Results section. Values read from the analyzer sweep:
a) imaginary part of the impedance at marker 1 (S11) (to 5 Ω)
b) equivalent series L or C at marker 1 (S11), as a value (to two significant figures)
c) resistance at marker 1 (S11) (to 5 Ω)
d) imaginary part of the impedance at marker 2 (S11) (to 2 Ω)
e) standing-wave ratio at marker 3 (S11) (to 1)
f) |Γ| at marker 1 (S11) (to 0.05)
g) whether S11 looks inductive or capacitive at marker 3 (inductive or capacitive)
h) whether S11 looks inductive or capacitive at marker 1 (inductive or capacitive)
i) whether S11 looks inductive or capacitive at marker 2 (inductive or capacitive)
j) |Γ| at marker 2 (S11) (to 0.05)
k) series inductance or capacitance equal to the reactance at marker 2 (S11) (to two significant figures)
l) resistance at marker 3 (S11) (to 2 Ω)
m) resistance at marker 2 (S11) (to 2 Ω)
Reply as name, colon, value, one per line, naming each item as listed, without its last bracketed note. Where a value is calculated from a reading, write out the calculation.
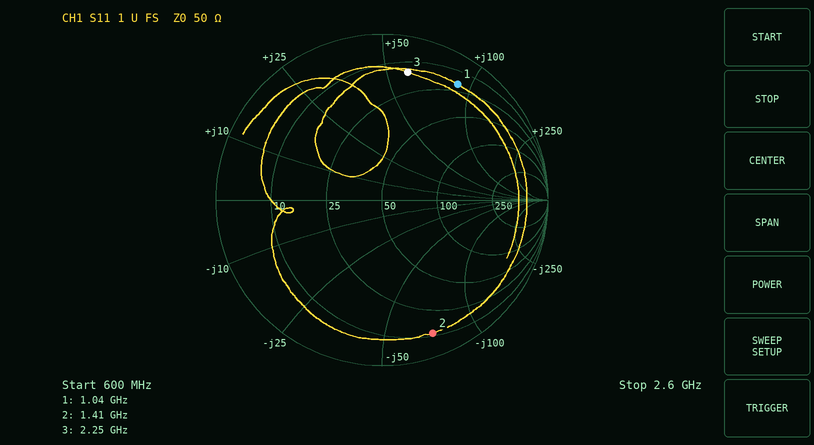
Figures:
imaginary part of the impedance at marker 1 (S11): +90 Ω
equivalent series L or C at marker 1 (S11), as a value: L = 90 Ω/(2π × 1.04 GHz) ≈ 14 nH
resistance at marker 1 (S11): 20 Ω
imaginary part of the impedance at marker 2 (S11): -72 Ω
standing-wave ratio at marker 3 (S11): 8
|Γ| at marker 1 (S11): 0.85
whether S11 looks inductive or capacitive at marker 3: inductive
whether S11 looks inductive or capacitive at marker 1: inductive
whether S11 looks inductive or capacitive at marker 2: capacitive
|Γ| at marker 2 (S11): 0.85
series inductance or capacitance equal to the reactance at marker 2 (S11): C = 1/(2π × 1.41 GHz × 72 Ω) ≈ 1.6 pF
resistance at marker 3 (S11): 14 Ω
resistance at marker 2 (S11): 12 Ω
